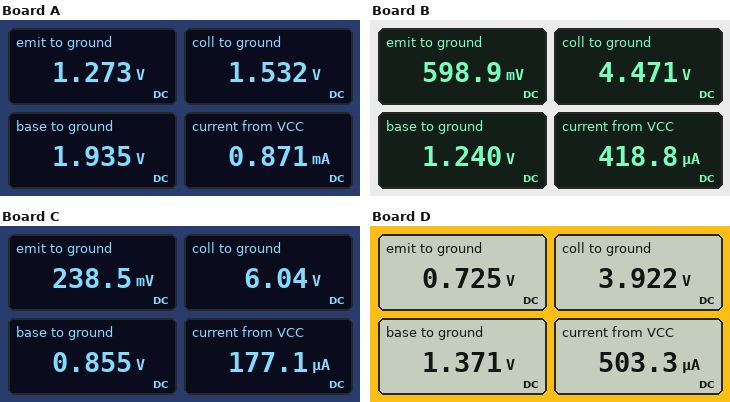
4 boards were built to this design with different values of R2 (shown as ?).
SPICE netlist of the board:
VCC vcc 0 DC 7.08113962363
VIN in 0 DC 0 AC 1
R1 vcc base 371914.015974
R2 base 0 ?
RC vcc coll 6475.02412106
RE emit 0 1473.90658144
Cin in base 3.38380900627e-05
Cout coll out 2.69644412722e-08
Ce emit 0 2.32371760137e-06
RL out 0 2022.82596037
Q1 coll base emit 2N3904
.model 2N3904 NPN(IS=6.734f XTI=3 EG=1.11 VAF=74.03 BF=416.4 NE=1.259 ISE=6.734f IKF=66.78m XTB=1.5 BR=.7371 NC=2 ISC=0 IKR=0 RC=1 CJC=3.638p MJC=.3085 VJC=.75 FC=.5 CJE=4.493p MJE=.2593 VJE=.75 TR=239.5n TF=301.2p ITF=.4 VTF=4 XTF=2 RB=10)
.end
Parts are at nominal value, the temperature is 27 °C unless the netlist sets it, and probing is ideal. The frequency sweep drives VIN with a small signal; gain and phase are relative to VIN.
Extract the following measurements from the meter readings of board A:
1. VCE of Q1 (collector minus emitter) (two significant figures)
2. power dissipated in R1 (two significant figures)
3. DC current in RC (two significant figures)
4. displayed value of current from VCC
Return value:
260 mV
71 µW
860 µA
0.871 mA
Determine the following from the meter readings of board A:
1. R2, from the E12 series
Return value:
270 kΩ
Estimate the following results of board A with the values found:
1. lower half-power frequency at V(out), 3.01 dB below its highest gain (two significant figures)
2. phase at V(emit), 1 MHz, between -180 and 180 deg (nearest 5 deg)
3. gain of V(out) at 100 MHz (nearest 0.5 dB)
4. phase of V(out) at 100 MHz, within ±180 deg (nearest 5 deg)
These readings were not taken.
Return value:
2.5 kHz
-90 deg
17.5 dB
90 deg
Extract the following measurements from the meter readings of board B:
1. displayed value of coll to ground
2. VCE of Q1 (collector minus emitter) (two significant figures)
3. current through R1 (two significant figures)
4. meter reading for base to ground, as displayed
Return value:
4.471 V
3.9 V
16 µA
1.240 V
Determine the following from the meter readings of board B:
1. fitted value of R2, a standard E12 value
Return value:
100 kΩ
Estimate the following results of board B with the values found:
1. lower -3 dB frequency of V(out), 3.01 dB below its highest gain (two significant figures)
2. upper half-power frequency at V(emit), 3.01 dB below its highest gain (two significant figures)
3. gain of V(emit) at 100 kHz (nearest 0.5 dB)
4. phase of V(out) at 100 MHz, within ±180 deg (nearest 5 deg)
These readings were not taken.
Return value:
1.4 kHz
1.1 kHz
-39.5 dB
105 deg
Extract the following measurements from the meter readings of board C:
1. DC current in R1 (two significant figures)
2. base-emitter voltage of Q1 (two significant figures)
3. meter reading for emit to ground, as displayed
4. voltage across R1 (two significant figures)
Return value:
17 µA
620 mV
238.5 mV
6.2 V
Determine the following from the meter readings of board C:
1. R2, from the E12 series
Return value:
56 kΩ
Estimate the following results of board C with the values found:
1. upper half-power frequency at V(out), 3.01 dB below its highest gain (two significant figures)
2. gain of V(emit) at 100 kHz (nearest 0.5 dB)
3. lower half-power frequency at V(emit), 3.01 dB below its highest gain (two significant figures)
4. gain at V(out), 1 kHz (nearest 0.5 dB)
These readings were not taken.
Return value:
51 MHz
-47.5 dB
120 mHz
17.0 dB
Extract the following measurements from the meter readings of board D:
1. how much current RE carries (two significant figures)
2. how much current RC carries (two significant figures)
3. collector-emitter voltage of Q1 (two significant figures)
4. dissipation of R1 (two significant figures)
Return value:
490 µA
490 µA
3.2 V
88 µW
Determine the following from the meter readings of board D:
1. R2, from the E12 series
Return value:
120 kΩ
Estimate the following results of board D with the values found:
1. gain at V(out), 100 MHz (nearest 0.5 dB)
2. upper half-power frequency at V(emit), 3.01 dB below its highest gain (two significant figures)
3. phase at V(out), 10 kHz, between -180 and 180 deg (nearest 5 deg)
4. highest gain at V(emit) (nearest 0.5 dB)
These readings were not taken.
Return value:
20.0 dB
1.3 kHz
-170 deg
-0.5 dB
